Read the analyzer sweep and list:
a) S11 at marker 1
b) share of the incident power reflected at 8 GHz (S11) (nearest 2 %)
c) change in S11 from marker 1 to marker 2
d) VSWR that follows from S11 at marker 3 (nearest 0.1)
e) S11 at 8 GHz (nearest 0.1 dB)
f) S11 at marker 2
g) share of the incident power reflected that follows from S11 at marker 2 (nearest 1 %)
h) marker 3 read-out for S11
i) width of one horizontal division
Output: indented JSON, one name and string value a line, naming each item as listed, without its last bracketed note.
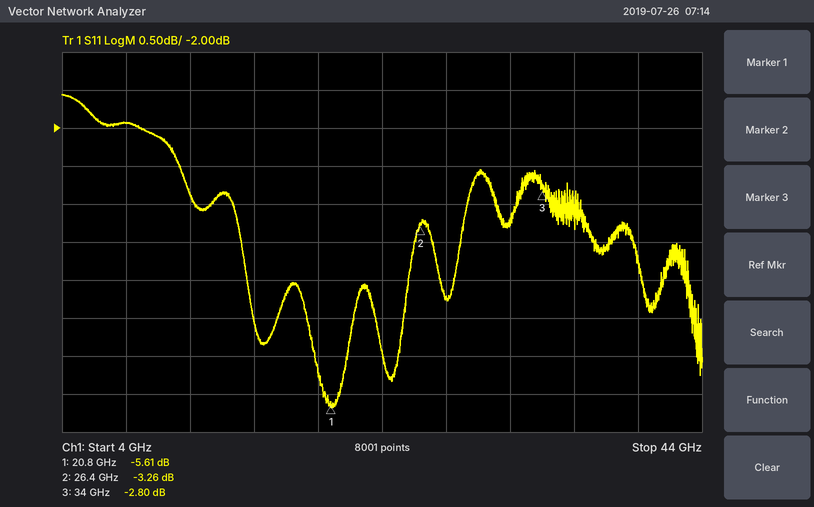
{
  "S11 at marker 1": "-5.61 dB",
  "share of the incident power reflected at 8 GHz (S11)": "64 %",
  "change in S11 from marker 1 to marker 2": "2.35 dB",
  "VSWR that follows from S11 at marker 3": "6.3",
  "S11 at 8 GHz": "-1.9 dB",
  "S11 at marker 2": "-3.26 dB",
  "share of the incident power reflected that follows from S11 at marker 2": "47 %",
  "marker 3 read-out for S11": "-2.80 dB",
  "width of one horizontal division": "4 GHz"
}
